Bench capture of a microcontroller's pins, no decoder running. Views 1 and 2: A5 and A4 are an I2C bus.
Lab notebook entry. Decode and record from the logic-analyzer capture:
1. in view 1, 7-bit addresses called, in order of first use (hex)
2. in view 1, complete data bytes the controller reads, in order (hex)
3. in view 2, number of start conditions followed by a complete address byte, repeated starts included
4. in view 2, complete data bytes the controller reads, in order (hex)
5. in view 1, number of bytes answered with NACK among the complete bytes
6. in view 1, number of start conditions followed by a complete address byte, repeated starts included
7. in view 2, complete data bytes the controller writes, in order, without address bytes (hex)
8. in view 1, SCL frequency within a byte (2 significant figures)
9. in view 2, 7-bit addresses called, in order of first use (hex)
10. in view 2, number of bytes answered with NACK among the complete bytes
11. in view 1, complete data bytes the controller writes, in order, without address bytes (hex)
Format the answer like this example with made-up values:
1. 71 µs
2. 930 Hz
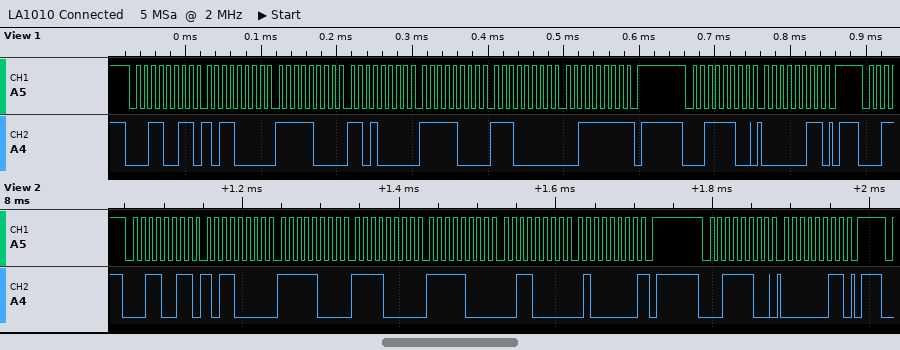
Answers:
1. 0x19 0x1E
2. B0 F8 D0 F8 E0 3F
3. 2
4. B0 F8 F0 F8 30 40
5. 1
6. 2
7. 03
8. 100 kHz
9. 0x19 0x1E
10. 1
11. 03
